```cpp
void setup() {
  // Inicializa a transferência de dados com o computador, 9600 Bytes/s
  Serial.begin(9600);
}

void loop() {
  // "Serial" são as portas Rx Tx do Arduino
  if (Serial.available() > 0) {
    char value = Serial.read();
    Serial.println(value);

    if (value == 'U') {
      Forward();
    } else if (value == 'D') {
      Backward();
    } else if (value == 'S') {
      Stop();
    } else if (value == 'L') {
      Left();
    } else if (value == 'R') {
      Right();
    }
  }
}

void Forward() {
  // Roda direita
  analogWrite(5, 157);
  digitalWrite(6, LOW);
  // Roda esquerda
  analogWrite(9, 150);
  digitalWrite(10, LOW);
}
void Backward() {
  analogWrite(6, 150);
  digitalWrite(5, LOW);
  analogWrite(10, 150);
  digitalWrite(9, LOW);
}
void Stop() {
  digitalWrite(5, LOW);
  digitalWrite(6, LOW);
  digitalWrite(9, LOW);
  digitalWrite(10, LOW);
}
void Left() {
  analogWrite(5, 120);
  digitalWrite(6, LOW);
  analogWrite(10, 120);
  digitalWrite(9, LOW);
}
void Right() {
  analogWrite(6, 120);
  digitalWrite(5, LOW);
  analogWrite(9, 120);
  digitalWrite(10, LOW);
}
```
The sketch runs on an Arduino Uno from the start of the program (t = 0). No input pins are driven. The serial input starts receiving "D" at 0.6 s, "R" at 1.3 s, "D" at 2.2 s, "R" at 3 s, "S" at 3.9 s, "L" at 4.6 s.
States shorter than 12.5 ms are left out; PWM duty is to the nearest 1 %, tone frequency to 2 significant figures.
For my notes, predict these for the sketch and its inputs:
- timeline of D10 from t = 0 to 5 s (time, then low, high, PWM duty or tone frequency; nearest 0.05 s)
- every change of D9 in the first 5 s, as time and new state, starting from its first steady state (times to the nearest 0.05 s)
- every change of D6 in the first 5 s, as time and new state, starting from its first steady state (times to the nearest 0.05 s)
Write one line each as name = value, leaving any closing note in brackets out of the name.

timeline of D10 from t = 0 to 5 s = 0.6 s PWM 59 %; 1.3 s low; 2.2 s PWM 59 %; 3 s low; 4.6 s PWM 47 %
every change of D9 in the first 5 s, as time and new state, starting from its first steady state = 1.3 s PWM 47 %; 2.2 s low; 3 s PWM 47 %; 3.9 s low
every change of D6 in the first 5 s, as time and new state, starting from its first steady state = 0.6 s PWM 59 %; 1.3 s PWM 47 %; 2.2 s PWM 59 %; 3 s PWM 47 %; 3.9 s low
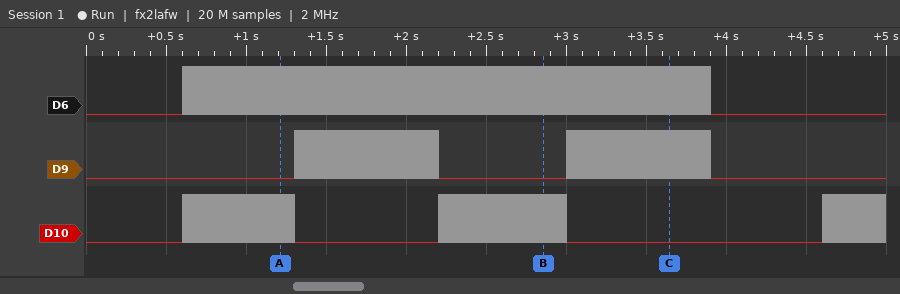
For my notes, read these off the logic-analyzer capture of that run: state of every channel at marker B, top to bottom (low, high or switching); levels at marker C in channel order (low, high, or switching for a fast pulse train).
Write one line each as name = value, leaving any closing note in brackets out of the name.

state of every channel at marker B, top to bottom = D6 switching, D9 low, D10 switching
levels at marker C in channel order = D6 switching, D9 switching, D10 low
